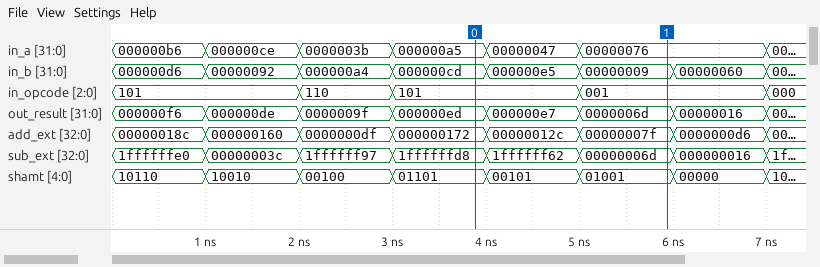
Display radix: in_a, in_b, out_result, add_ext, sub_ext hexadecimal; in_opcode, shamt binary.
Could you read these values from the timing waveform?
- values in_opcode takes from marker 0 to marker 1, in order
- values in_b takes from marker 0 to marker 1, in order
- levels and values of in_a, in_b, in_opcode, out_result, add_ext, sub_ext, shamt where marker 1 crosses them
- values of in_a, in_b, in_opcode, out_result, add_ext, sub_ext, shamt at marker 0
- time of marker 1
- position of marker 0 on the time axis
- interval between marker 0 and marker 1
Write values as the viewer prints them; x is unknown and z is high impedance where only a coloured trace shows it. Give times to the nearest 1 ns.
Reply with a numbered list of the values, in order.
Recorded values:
1. 101, 001
2. 000000cd, 000000e5, 00000009
3. in_a=00000076, in_b=00000009, in_opcode=001, out_result=0000006d, add_ext=00000007f, sub_ext=00000006d, shamt=01001
4. in_a=000000a5, in_b=000000cd, in_opcode=101, out_result=000000ed, add_ext=000000172, sub_ext=1ffffffd8, shamt=01101
5. 6 ns
6. 4 ns
7. 2 ns
